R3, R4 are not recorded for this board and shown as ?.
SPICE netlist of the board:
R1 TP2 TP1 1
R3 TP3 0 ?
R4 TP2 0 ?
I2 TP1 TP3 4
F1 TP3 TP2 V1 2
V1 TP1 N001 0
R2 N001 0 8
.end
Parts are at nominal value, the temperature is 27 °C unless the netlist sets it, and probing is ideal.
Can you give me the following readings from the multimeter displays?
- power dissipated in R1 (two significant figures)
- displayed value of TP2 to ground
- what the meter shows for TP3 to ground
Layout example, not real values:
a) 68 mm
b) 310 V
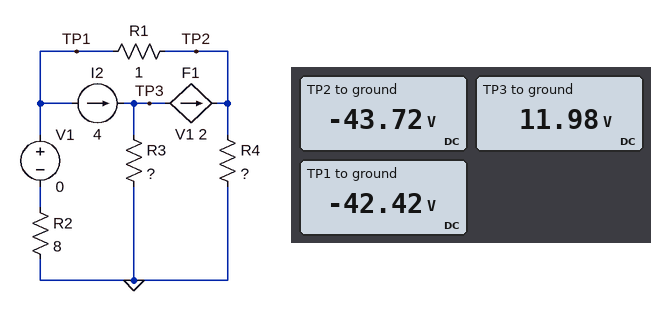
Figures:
a) 1.7 W
b) -43.72 V
c) 11.98 V
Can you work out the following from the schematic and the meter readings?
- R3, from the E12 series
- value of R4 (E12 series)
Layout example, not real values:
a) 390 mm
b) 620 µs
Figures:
a) 0.82 Ω
b) 4.7 Ω
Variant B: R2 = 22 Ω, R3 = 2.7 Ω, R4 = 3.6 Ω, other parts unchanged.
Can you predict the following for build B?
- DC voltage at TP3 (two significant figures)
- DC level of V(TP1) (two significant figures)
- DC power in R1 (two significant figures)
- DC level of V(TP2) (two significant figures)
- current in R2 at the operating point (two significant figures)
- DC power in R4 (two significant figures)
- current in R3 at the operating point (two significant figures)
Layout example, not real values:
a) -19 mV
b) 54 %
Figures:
a) 16 V
b) -21 V
c) 9.3 W
d) -18 V
e) 950 mA
f) 88 W
g) 5.9 A
